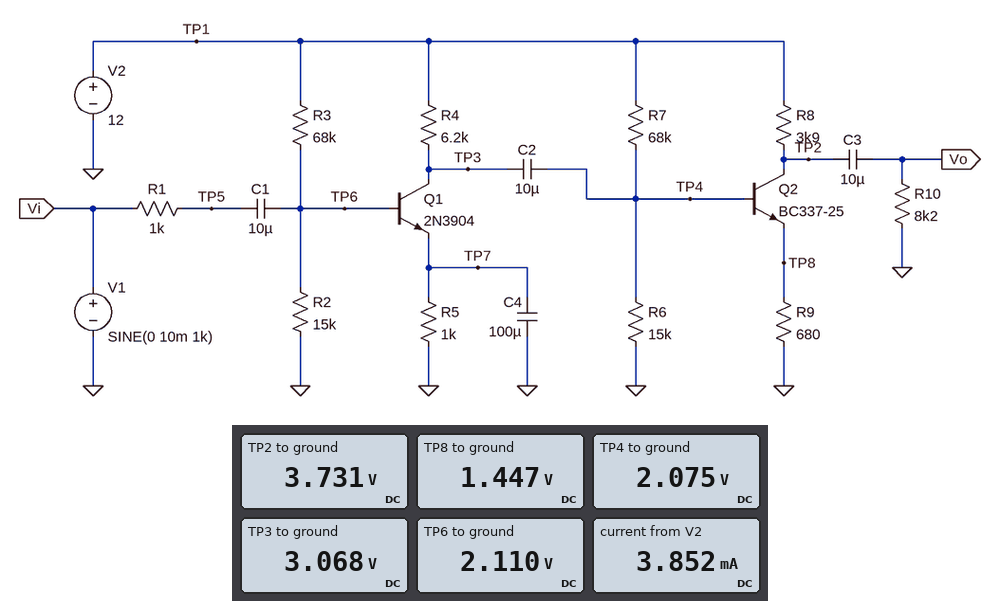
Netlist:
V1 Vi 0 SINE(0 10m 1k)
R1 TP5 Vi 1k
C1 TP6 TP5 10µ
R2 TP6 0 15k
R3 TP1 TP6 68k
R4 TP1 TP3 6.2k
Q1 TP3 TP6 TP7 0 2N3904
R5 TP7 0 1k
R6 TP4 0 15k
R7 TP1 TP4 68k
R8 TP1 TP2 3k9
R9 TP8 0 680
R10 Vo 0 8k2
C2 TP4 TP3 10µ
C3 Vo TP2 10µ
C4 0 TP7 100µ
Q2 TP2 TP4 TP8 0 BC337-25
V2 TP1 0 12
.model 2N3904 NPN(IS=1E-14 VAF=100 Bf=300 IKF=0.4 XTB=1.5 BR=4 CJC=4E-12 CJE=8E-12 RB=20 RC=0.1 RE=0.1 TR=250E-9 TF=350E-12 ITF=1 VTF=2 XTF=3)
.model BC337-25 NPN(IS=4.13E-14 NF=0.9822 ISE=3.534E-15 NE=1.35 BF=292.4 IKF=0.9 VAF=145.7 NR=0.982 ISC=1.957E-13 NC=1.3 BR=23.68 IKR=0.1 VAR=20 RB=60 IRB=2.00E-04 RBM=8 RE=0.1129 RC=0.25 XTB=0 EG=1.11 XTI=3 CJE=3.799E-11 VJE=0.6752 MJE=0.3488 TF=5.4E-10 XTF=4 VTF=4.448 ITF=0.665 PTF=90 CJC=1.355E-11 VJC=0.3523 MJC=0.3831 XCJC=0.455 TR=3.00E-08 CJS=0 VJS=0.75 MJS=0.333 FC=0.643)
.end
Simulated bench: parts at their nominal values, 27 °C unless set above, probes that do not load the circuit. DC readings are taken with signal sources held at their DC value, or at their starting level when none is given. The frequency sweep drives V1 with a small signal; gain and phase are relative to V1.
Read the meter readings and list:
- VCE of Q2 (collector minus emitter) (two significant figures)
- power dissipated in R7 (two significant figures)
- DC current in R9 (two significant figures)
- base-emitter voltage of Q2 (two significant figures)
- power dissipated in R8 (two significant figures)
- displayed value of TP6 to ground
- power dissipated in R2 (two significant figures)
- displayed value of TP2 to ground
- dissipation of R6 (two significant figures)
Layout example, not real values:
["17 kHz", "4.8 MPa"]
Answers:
["2.3 V", "1.4 mW", "2.1 mA", "630 mV", "18 mW", "2.110 V", "300 µW", "3.731 V", "290 µW"]
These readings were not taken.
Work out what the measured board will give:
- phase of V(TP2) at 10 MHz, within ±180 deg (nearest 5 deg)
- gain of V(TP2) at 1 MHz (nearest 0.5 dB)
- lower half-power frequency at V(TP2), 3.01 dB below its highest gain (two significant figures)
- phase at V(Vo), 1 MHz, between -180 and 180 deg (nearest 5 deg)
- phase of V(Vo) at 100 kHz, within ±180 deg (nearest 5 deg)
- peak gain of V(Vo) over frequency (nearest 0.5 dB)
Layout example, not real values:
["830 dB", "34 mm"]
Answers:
["-165 deg", "43.0 dB", "75 Hz", "-85 deg", "-25 deg", "56.0 dB"]
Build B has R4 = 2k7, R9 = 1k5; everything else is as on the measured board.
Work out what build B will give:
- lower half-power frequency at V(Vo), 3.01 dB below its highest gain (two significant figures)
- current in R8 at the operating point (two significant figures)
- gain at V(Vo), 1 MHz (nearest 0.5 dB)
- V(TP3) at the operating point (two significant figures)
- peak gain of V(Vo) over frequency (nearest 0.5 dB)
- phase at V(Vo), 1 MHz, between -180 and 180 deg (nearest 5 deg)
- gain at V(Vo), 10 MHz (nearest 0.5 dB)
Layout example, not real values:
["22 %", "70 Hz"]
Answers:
["77 Hz", "1.0 mA", "39.0 dB", "8.1 V", "44.0 dB", "-65 deg", "19.0 dB"]
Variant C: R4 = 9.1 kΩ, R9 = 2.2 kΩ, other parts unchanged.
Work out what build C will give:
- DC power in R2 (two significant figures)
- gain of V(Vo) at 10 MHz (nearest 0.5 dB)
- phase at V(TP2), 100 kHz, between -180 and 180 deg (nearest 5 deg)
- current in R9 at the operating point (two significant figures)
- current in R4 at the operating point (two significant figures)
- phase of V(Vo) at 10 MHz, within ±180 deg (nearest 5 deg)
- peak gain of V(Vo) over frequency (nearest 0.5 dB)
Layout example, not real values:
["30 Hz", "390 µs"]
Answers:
["230 µW", "-30.0 dB", "-30 deg", "700 µA", "1.2 mA", "145 deg", "1.5 dB"]
